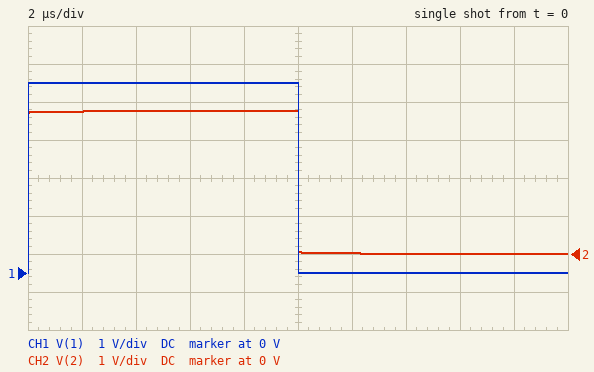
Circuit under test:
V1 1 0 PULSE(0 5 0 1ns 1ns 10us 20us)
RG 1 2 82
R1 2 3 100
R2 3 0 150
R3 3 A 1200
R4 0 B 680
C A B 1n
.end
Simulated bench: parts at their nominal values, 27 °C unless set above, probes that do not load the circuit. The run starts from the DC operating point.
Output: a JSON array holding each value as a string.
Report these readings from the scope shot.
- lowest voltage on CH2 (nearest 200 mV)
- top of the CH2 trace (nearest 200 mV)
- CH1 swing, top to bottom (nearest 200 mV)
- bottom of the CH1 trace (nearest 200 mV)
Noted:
["0 V", "3.8 V", "5.0 V", "0 V"]
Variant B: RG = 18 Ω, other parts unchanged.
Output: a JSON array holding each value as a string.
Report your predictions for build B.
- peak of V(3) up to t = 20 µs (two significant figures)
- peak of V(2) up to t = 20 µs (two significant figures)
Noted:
["2.8 V", "4.7 V"]
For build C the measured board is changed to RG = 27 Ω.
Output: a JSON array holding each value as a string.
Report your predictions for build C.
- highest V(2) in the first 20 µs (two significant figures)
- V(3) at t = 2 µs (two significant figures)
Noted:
["4.5 V", "2.7 V"]
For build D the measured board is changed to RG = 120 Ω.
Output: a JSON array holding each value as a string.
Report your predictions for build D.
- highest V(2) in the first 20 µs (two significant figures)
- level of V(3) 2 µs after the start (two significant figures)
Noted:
["3.4 V", "2.0 V"]
